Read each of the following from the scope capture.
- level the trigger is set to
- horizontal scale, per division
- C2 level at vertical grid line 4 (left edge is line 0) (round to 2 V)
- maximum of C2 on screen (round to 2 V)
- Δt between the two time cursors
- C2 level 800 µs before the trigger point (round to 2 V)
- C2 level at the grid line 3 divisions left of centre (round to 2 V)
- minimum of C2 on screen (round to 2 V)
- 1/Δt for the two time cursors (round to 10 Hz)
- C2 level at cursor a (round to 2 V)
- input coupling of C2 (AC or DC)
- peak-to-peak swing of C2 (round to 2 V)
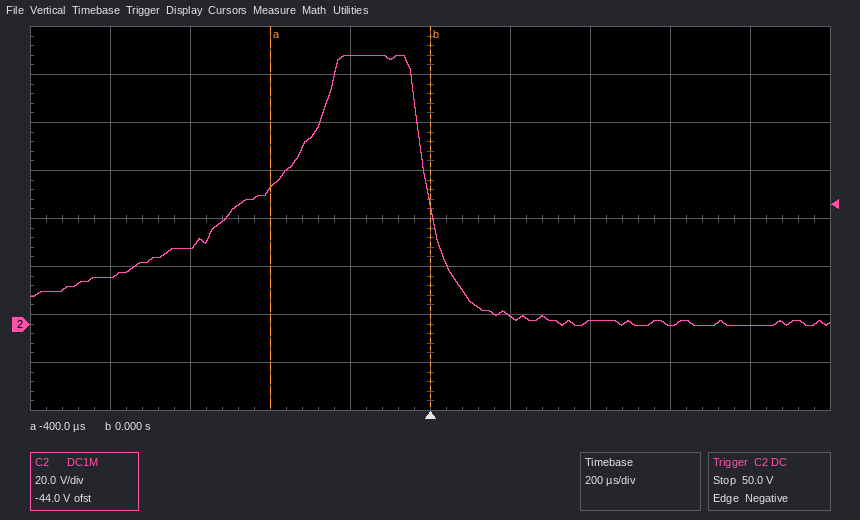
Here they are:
50.0 V
200 µs
112 V
112 V
400 µs
20 V
32 V
0 V
2.50 kHz
56 V
DC
112 V
